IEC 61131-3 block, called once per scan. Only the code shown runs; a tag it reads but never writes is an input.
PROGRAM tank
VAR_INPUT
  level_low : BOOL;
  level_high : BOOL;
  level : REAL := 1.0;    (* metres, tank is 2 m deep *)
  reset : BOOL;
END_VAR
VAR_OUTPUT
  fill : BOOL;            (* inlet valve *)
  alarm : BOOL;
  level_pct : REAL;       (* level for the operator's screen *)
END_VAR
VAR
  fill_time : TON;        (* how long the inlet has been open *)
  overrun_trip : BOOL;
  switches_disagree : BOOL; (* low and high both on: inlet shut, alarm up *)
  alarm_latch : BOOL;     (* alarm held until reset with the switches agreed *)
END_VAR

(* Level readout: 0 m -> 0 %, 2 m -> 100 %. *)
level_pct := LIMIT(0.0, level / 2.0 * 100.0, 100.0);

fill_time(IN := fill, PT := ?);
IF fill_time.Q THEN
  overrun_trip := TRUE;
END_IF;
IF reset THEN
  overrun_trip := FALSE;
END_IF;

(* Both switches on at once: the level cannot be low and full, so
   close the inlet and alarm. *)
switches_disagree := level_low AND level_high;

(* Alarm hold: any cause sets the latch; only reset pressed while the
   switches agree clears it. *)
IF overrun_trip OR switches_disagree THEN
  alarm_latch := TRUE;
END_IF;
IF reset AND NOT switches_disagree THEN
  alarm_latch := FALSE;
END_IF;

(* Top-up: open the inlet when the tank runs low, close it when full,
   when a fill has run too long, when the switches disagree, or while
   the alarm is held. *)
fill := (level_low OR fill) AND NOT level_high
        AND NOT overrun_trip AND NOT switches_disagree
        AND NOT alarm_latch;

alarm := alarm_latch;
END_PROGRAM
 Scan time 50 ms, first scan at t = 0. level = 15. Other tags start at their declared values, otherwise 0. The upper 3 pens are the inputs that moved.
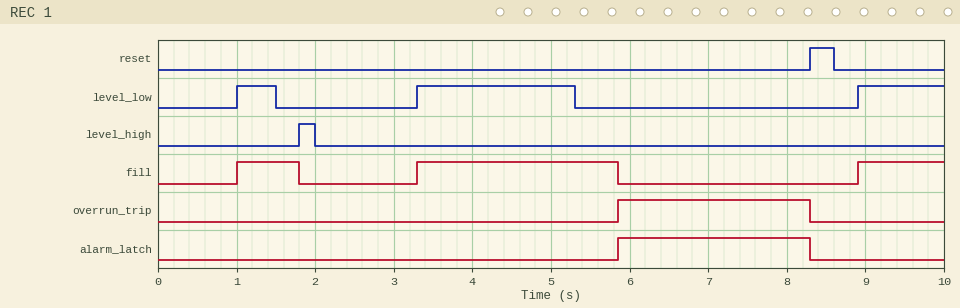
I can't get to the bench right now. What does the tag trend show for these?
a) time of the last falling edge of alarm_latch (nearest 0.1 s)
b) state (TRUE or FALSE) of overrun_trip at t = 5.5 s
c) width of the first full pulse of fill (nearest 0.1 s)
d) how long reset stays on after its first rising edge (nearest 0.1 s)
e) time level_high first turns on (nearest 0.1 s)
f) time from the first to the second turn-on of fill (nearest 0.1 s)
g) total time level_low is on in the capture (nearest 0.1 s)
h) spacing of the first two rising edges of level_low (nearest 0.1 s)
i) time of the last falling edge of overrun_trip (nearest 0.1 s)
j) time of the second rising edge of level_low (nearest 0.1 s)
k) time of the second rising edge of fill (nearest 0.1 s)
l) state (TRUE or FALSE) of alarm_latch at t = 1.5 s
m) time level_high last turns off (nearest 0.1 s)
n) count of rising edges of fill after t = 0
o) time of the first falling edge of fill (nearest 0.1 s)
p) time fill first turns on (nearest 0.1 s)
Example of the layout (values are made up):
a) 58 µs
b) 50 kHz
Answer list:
a) 8.3 s
b) FALSE
c) 0.8 s
d) 0.3 s
e) 1.8 s
f) 2.3 s
g) 3.6 s
h) 2.3 s
i) 8.3 s
j) 3.3 s
k) 3.3 s
l) FALSE
m) 2.0 s
n) 3
o) 1.8 s
p) 1.0 s
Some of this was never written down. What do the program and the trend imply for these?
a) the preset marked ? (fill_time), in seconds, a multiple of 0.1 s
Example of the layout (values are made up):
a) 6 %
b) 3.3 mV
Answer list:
a) 2.5 s
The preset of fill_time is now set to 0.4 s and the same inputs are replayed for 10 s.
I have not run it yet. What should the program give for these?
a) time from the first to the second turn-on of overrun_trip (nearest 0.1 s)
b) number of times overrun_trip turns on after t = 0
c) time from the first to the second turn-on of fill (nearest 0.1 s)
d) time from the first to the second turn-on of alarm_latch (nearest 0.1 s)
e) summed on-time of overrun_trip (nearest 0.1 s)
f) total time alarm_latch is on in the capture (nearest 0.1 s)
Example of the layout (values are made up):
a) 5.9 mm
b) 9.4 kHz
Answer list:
a) 7.9 s
b) 2
c) 7.9 s
d) 7.9 s
e) 7.5 s
f) 7.5 s
